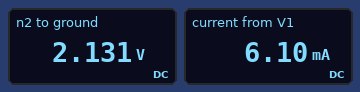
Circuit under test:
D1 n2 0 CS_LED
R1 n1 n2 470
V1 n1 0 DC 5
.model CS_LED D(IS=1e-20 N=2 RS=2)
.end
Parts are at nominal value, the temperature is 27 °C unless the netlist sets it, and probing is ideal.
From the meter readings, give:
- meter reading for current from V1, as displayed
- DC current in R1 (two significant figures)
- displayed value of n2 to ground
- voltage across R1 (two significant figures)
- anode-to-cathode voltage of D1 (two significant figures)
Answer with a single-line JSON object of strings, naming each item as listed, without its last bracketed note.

{"meter reading for current from V1, as displayed": "6.10 mA", "DC current in R1": "6.1 mA", "displayed value of n2 to ground": "2.131 V", "voltage across R1": "2.9 V", "anode-to-cathode voltage of D1": "2.1 V"}
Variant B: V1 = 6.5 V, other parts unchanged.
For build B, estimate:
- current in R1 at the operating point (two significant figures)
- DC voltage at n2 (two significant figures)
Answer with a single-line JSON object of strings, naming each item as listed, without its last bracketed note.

{"current in R1 at the operating point": "9.2 mA", "DC voltage at n2": "2.2 V"}
